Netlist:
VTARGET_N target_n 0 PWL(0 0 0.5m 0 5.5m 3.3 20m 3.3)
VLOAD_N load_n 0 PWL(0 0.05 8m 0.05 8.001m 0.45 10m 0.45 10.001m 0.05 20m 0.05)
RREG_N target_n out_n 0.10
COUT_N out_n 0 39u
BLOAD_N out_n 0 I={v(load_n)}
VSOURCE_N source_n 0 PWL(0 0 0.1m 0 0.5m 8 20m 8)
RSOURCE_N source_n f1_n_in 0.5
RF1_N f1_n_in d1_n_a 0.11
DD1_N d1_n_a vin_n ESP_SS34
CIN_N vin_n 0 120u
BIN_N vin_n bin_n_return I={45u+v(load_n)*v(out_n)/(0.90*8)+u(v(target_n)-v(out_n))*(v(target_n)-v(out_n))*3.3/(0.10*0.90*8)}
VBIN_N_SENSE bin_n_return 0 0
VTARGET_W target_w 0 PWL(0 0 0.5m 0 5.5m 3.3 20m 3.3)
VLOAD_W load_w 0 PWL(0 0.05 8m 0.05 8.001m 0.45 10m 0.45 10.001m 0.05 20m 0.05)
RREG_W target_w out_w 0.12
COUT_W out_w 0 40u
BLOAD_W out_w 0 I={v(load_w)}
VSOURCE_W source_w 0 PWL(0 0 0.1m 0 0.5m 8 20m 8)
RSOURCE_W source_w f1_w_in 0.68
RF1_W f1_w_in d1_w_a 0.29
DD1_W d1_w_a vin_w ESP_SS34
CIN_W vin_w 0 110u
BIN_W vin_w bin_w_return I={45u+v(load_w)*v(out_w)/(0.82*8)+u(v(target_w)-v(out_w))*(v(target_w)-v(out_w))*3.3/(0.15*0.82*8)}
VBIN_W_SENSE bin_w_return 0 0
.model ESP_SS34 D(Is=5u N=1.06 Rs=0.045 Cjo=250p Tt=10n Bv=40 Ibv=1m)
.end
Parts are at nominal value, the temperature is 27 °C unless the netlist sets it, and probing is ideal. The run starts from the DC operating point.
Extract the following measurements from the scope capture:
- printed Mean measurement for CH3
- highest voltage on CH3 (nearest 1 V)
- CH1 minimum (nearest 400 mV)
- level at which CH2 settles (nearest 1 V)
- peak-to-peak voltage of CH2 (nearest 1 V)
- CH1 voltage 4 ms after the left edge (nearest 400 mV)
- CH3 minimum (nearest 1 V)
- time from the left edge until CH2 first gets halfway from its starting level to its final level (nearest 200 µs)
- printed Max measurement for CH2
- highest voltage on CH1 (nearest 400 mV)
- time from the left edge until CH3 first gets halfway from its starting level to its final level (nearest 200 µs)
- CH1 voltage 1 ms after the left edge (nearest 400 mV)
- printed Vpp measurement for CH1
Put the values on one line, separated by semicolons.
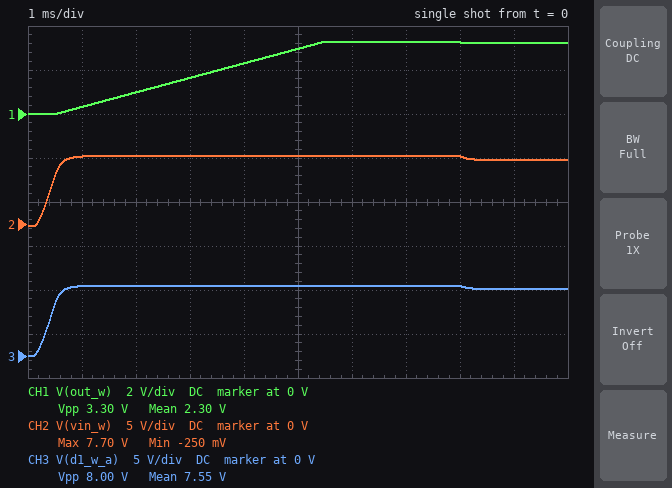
7.55 V; 8 V; 0 V; 7 V; 8 V; 2.4 V; 0 V; 400 µs; 7.70 V; 3.2 V; 400 µs; 400 mV; 3.30 V
